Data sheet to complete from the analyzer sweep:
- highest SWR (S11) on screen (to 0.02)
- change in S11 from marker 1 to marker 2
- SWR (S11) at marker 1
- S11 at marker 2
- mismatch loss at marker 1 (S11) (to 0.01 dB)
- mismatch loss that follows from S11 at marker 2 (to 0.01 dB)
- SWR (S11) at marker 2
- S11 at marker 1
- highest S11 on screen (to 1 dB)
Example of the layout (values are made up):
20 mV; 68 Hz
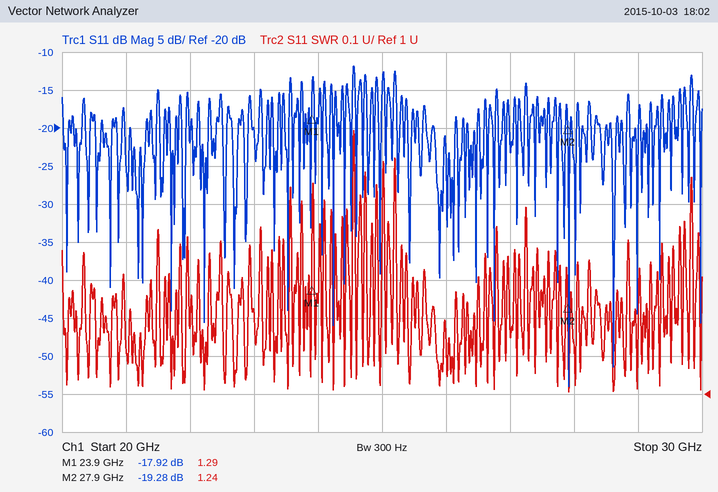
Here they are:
1.70; -1.36 dB; 1.29; -19.28 dB; 0.07 dB; 0.05 dB; 1.24; -17.92 dB; -12 dB
